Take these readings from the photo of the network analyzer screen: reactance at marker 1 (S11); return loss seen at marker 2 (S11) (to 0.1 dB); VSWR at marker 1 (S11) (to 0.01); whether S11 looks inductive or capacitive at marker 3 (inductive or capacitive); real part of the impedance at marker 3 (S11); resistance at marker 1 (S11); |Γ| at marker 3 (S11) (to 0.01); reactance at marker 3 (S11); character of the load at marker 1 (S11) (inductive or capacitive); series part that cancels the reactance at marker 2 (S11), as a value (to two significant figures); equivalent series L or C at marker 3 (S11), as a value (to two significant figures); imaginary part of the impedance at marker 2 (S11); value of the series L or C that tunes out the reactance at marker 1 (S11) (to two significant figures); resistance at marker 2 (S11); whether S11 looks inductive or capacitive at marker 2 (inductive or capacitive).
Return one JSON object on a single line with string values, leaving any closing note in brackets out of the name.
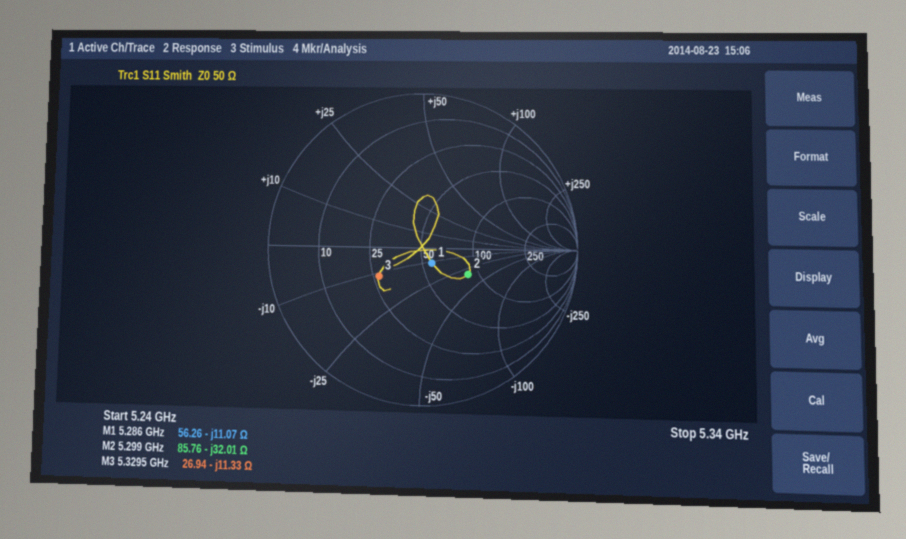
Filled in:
{"reactance at marker 1": "-11.07 Ω", "return loss seen at marker 2 (S11)": "9.3 dB", "VSWR at marker 1 (S11)": "1.27", "whether S11 looks inductive or capacitive at marker 3": "capacitive", "real part of the impedance at marker 3": "26.94 Ω", "resistance at marker 1": "56.26 Ω", "|Γ| at marker 3 (S11)": "0.33", "reactance at marker 3": "-11.33 Ω", "character of the load at marker 1 (S11)": "capacitive", "series part that cancels the reactance at marker 2 (S11), as a value": "960 pH", "equivalent series L or C at marker 3 (S11), as a value": "2.6 pF", "imaginary part of the impedance at marker 2": "-32.01 Ω", "value of the series L or C that tunes out the reactance at marker 1 (S11)": "330 pH", "resistance at marker 2": "85.76 Ω", "whether S11 looks inductive or capacitive at marker 2": "capacitive"}
